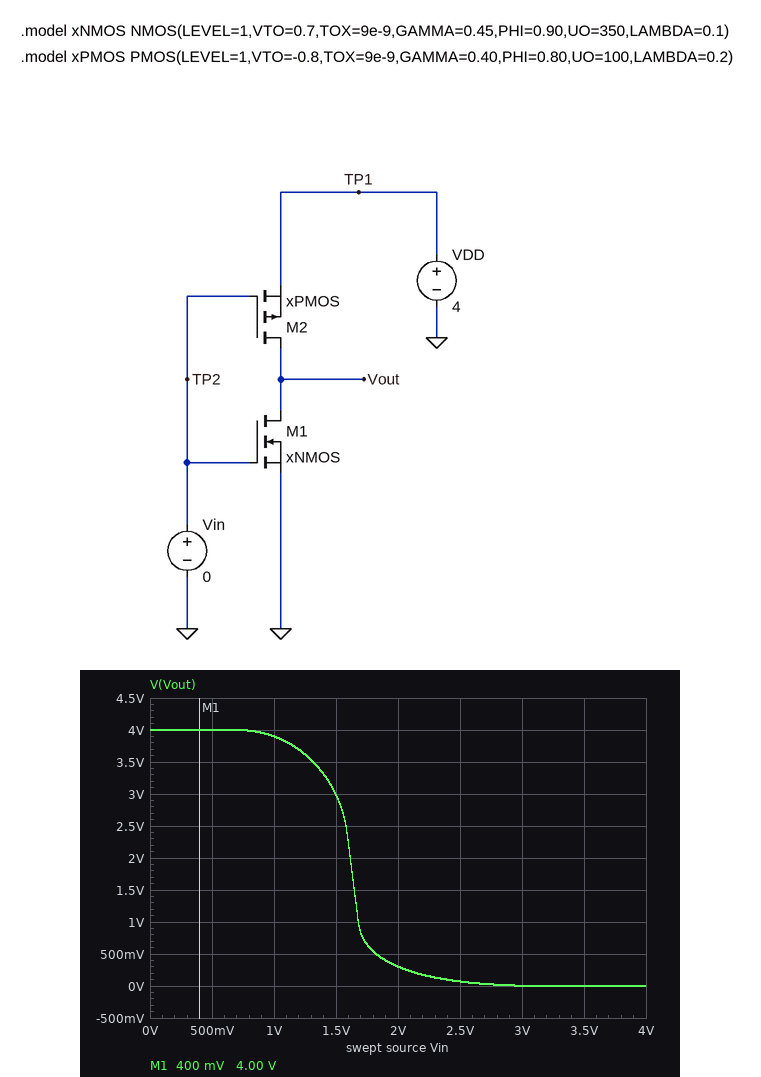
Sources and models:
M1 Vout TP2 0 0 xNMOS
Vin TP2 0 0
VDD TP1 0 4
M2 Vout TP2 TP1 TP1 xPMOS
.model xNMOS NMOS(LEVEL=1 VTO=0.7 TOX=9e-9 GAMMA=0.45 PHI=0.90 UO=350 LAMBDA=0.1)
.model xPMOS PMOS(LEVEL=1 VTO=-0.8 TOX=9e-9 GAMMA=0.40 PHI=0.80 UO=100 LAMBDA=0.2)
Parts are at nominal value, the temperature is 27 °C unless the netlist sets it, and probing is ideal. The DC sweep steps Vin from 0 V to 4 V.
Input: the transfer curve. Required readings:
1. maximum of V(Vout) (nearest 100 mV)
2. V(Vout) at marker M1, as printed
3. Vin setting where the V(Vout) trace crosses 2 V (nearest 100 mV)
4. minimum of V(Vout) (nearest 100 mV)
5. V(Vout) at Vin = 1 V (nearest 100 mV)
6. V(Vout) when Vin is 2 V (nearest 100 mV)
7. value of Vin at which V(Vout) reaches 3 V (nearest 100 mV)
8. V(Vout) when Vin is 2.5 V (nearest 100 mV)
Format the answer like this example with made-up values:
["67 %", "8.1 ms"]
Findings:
["4.0 V", "4.00 V", "1.6 V", "0 V", "3.9 V", "300 mV", "1.5 V", "100 mV"]
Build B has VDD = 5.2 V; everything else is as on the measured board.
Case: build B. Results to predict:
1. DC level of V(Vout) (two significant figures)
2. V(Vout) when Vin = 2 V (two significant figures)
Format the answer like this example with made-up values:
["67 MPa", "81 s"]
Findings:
["5.2 V", "3.2 V"]
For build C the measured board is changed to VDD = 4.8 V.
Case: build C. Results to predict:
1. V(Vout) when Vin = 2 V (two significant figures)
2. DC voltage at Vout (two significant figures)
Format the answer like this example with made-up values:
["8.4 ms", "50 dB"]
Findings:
["1.4 V", "4.8 V"]
